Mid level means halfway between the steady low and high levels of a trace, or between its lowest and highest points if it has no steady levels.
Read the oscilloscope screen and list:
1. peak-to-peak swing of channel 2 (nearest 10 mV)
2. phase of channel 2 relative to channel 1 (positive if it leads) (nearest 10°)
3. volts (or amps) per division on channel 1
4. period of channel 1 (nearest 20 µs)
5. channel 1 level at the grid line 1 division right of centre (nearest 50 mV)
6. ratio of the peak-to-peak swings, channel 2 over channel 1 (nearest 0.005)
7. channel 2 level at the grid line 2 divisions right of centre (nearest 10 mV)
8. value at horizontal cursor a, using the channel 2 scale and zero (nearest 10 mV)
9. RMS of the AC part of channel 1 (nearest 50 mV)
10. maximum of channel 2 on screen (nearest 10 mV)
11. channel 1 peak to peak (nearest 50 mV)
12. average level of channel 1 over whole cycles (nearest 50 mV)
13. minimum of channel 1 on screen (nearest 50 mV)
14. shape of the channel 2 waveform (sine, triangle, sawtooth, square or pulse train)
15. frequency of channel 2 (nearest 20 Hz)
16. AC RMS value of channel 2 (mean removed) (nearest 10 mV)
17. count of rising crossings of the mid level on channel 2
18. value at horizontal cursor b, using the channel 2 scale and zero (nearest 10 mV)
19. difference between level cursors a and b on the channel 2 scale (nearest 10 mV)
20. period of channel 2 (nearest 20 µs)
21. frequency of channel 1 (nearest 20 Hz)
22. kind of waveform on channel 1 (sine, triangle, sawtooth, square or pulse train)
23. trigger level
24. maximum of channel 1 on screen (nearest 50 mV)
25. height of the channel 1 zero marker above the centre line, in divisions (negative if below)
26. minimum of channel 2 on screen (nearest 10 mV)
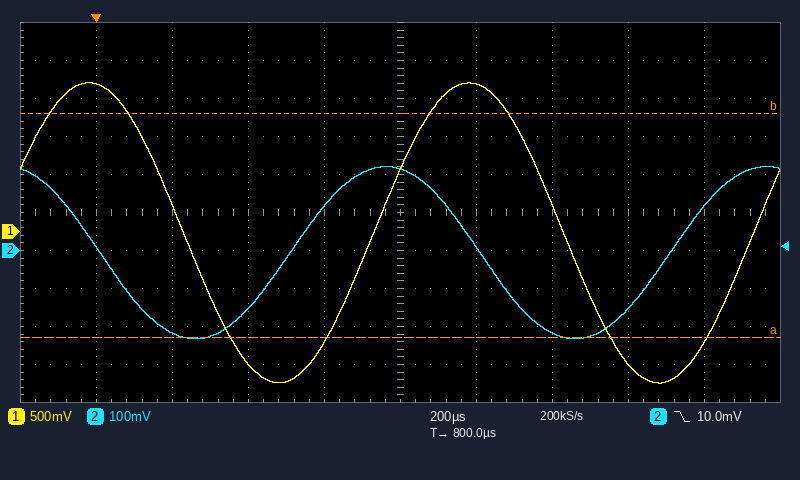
450 mV
+80°
500 mV
1.00 ms
1.95 V
0.115
-220 mV
-230 mV
1.40 V
220 mV
3.95 V
0 mV
-2.00 V
sine
1.00 kHz
160 mV
2
360 mV
590 mV
1.00 ms
1.00 kHz
sine
10.0 mV
1.95 V
-0.5 div
-230 mV
